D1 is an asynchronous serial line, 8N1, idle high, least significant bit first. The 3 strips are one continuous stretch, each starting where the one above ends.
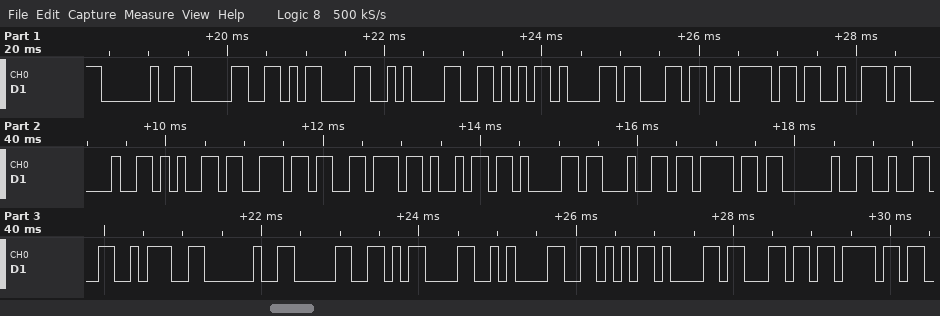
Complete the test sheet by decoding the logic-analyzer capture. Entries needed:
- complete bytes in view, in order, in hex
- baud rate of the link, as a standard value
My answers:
20 30 0D 0A 56 61 6C 6F 72 20 65 6E 76 69 61 64 6F 20 32 3A 20 30 0D 0A 56 61 6C 6F
9600 baud
